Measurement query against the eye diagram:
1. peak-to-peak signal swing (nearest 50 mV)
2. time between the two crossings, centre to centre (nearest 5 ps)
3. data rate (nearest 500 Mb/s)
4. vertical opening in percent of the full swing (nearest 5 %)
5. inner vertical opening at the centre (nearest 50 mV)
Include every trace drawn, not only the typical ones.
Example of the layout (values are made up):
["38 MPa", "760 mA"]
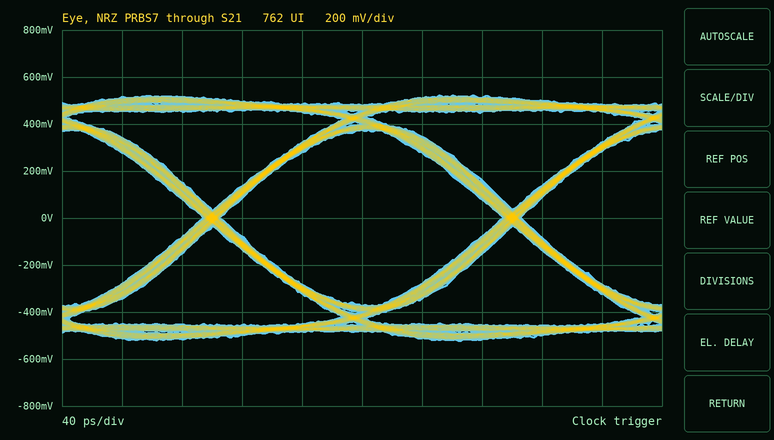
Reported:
["1.05 V", "200 ps", "5.0 Gb/s", "70 %", "750 mV"]
